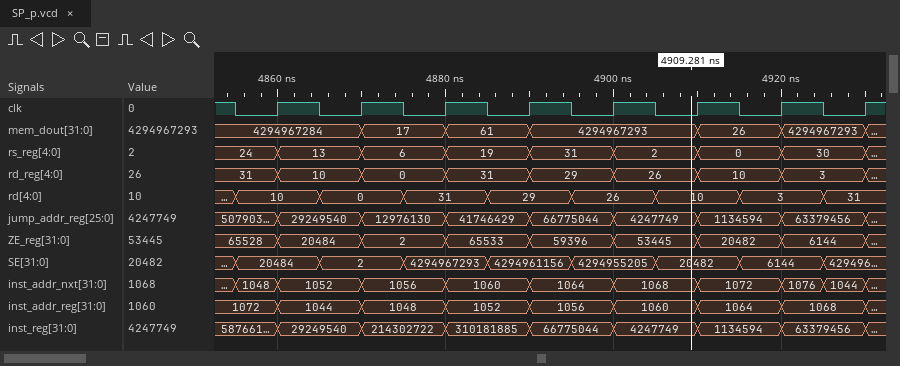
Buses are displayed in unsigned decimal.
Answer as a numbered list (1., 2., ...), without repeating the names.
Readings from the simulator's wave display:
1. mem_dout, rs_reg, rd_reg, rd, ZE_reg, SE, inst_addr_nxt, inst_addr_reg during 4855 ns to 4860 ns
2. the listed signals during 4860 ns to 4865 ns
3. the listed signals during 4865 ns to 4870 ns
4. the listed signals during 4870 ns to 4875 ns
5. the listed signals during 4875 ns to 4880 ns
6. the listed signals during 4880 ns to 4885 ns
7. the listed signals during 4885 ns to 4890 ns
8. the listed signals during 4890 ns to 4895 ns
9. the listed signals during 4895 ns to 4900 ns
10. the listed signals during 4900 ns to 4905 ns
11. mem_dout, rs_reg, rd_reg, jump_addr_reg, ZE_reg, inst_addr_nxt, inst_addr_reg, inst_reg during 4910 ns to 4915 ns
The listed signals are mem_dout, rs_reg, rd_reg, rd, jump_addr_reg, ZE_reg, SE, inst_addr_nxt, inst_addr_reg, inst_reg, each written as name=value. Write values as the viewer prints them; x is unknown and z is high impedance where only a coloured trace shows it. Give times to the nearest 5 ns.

1. mem_dout=4294967284, rs_reg=24, rd_reg=31, rd=10, ZE_reg=65528, SE=20484, inst_addr_nxt=1048, inst_addr_reg=1072
2. mem_dout=4294967284, rs_reg=13, rd_reg=10, rd=10, jump_addr_reg=29249540, ZE_reg=20484, SE=20484, inst_addr_nxt=1052, inst_addr_reg=1044, inst_reg=29249540
3. mem_dout=4294967284, rs_reg=13, rd_reg=10, rd=0, jump_addr_reg=29249540, ZE_reg=20484, SE=2, inst_addr_nxt=1052, inst_addr_reg=1044, inst_reg=29249540
4. mem_dout=17, rs_reg=6, rd_reg=0, rd=0, jump_addr_reg=12976130, ZE_reg=2, SE=2, inst_addr_nxt=1056, inst_addr_reg=1048, inst_reg=214302722
5. mem_dout=17, rs_reg=6, rd_reg=0, rd=31, jump_addr_reg=12976130, ZE_reg=2, SE=4294967293, inst_addr_nxt=1056, inst_addr_reg=1048, inst_reg=214302722
6. mem_dout=61, rs_reg=19, rd_reg=31, rd=31, jump_addr_reg=41746429, ZE_reg=65533, SE=4294967293, inst_addr_nxt=1060, inst_addr_reg=1052, inst_reg=310181885
7. mem_dout=61, rs_reg=19, rd_reg=31, rd=29, jump_addr_reg=41746429, ZE_reg=65533, SE=4294961156, inst_addr_nxt=1060, inst_addr_reg=1052, inst_reg=310181885
8. mem_dout=4294967293, rs_reg=31, rd_reg=29, rd=29, jump_addr_reg=66775044, ZE_reg=59396, SE=4294961156, inst_addr_nxt=1064, inst_addr_reg=1056, inst_reg=66775044
9. mem_dout=4294967293, rs_reg=31, rd_reg=29, rd=26, jump_addr_reg=66775044, ZE_reg=59396, SE=4294955205, inst_addr_nxt=1064, inst_addr_reg=1056, inst_reg=66775044
10. mem_dout=4294967293, rs_reg=2, rd_reg=26, rd=26, jump_addr_reg=4247749, ZE_reg=53445, SE=4294955205, inst_addr_nxt=1068, inst_addr_reg=1060, inst_reg=4247749
11. mem_dout=26, rs_reg=0, rd_reg=10, jump_addr_reg=1134594, ZE_reg=20482, inst_addr_nxt=1072, inst_addr_reg=1064, inst_reg=1134594
